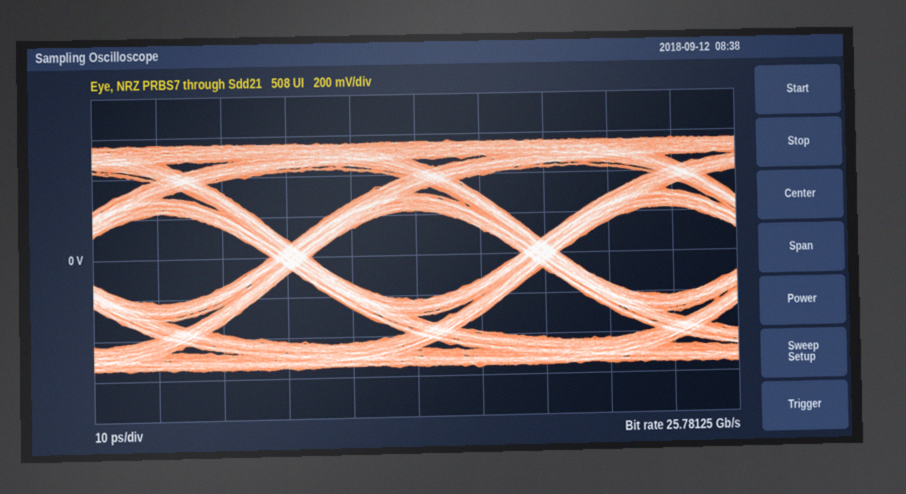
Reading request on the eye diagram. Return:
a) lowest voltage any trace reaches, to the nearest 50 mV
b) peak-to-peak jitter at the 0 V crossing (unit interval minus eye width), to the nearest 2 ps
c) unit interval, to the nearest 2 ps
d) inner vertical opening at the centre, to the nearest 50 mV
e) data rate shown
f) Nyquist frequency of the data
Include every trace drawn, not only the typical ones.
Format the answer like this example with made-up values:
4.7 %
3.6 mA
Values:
-550 mV
6 ps
38 ps
450 mV
25.78125 Gb/s
12.89062 GHz
